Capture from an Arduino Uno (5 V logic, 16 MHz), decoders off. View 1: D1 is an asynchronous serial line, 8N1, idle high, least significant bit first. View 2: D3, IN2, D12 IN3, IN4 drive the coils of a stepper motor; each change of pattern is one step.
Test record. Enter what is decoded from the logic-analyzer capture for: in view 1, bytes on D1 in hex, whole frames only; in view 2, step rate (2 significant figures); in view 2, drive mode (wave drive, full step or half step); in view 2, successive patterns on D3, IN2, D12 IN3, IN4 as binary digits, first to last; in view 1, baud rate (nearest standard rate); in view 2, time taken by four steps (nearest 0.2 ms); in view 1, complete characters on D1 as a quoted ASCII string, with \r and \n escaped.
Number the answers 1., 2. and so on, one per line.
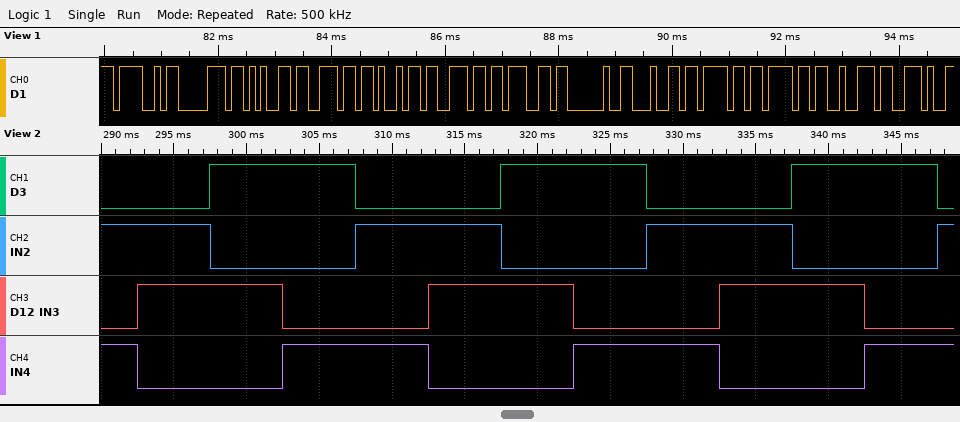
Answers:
1. 0x4F 0x70 0x65 0x6E 0x69 0x6E 0x67 0x20 0x64 0x6F 0x6F 0x72 0x2E
2. 200 steps/s
3. full step
4. 0101 0110 1010 1001 0101 0110 1010 1001 0101 0110 1010 1001 0101
5. 9600 baud
6. 20.0 ms
7. "Opening door."
